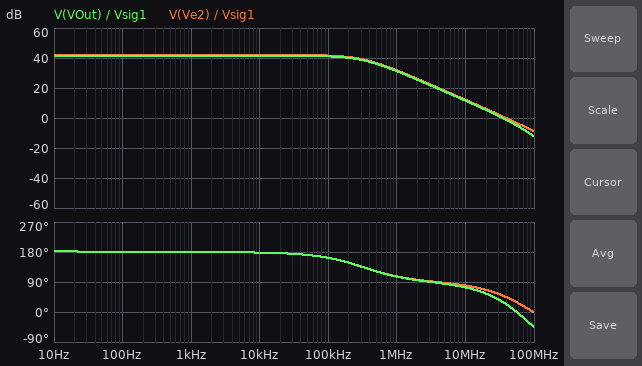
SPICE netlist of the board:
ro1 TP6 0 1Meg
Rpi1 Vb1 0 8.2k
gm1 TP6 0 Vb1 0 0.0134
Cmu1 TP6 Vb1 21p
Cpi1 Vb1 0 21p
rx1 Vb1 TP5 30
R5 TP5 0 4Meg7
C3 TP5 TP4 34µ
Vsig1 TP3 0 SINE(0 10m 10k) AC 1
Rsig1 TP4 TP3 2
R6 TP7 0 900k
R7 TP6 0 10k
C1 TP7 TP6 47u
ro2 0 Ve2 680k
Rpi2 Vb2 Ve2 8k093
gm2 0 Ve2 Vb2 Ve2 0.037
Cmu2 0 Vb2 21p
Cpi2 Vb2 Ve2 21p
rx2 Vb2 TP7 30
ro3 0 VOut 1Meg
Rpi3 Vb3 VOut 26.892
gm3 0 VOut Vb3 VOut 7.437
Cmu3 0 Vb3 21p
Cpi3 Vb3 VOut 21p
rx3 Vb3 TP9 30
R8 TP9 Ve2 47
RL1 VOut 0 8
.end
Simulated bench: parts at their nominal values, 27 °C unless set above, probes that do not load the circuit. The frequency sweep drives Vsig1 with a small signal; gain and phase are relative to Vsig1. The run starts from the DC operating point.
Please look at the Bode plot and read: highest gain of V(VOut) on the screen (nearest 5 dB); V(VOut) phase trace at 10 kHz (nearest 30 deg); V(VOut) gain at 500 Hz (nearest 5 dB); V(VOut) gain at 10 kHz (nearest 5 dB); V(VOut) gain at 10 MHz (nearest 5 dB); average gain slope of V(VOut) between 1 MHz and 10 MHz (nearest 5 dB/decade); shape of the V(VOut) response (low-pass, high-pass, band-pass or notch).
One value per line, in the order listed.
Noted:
40 dB
180 deg
40 dB
40 dB
10 dB
-20 dB/decade
low-pass
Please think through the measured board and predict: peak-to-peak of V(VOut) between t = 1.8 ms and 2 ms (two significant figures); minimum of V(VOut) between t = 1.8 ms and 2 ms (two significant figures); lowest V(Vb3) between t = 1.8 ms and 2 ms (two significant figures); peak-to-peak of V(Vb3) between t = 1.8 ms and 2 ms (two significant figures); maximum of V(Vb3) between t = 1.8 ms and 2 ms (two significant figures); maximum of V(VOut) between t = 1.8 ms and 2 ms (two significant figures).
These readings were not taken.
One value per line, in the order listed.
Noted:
2.4 V
-1.2 V
-1.2 V
2.4 V
1.2 V
1.2 V
